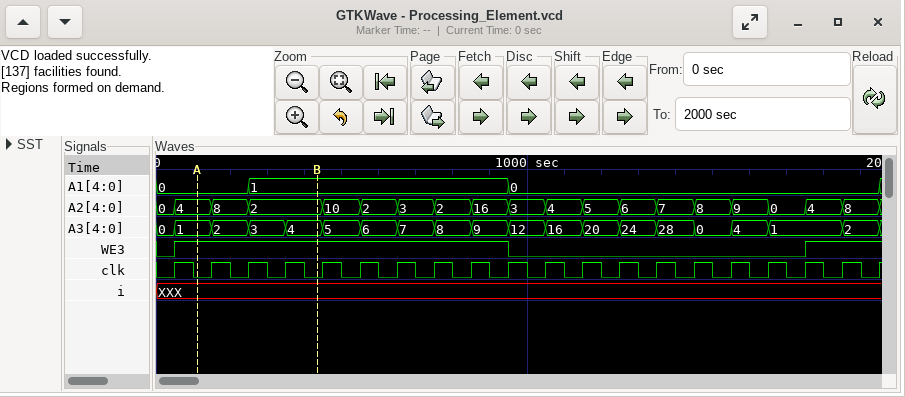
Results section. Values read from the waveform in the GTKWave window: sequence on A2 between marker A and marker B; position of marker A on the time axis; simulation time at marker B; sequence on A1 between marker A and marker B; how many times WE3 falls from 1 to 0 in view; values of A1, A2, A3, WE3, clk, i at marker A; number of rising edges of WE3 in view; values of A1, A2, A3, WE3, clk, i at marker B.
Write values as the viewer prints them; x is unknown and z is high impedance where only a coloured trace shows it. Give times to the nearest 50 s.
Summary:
4, 8, 2
100 s
450 s
0, 1
1
A1=0, A2=4, A3=1, WE3=1, clk=0, i=XXX
2
A1=1, A2=2, A3=4, WE3=1, clk=0, i=XXX
